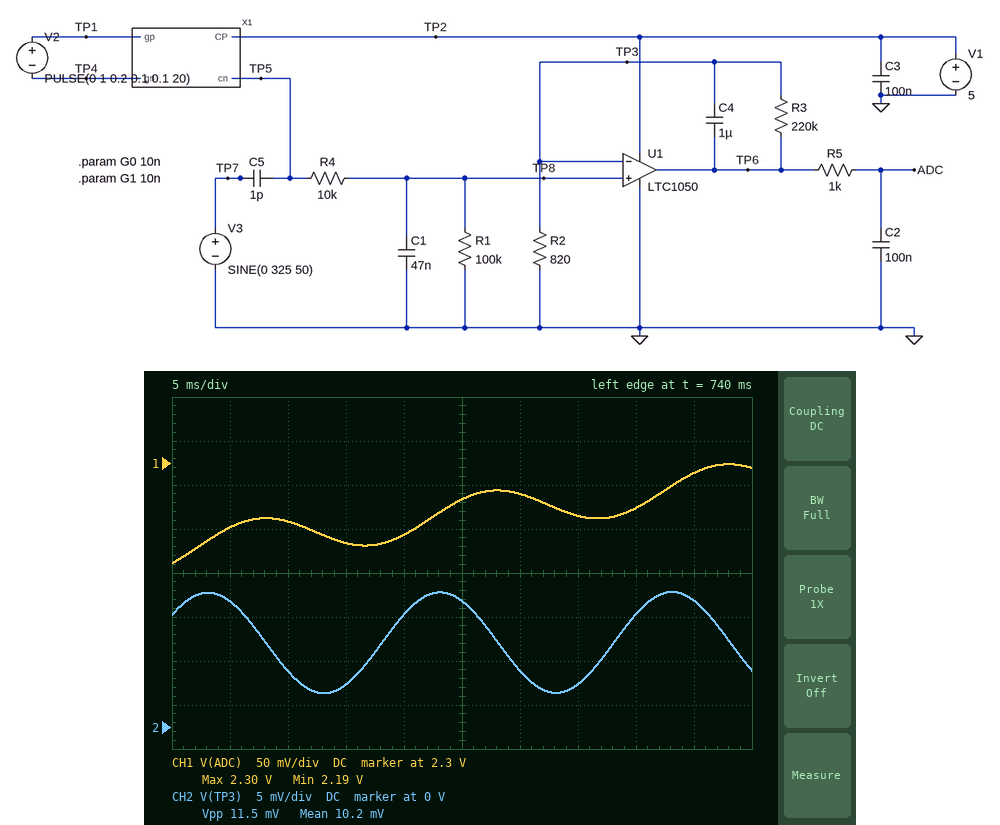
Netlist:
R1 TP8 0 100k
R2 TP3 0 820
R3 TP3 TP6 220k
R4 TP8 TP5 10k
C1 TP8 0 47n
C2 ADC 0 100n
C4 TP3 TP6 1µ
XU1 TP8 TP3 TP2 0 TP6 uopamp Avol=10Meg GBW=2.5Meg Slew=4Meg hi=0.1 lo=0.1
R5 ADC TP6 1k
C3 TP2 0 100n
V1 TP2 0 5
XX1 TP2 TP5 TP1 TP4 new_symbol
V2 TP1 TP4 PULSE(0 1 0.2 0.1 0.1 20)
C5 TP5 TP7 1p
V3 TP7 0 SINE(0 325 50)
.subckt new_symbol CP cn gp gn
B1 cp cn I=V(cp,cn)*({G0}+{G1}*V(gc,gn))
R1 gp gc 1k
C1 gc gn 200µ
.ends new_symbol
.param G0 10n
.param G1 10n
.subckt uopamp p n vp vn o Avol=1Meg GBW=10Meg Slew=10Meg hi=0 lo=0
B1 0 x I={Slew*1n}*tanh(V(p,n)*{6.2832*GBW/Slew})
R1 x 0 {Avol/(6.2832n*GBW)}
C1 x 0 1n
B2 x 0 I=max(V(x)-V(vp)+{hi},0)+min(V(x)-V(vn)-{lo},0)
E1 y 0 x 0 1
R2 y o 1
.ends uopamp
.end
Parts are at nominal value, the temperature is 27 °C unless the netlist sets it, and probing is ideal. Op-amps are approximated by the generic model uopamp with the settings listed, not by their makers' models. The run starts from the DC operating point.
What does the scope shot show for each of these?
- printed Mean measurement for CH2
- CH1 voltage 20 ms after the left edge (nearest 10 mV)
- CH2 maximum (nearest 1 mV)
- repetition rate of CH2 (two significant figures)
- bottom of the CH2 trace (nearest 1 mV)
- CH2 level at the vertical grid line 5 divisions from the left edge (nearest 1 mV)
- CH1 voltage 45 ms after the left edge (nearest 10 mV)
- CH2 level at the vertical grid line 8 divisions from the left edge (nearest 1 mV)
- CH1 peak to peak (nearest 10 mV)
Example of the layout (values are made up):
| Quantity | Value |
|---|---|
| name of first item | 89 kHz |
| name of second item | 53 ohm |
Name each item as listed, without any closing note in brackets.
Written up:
| Quantity | Value |
|---|---|
| printed Mean measurement for CH2 | 10.2 mV |
| CH1 voltage 20 ms after the left edge | 2.22 V |
| CH2 maximum | 15 mV |
| repetition rate of CH2 | 50 Hz |
| bottom of the CH2 trace | 4 mV |
| CH2 level at the vertical grid line 5 divisions from the left edge | 14 mV |
| CH1 voltage 45 ms after the left edge | 2.29 V |
| CH2 level at the vertical grid line 8 divisions from the left edge | 13 mV |
| CH1 peak to peak | 110 mV |
